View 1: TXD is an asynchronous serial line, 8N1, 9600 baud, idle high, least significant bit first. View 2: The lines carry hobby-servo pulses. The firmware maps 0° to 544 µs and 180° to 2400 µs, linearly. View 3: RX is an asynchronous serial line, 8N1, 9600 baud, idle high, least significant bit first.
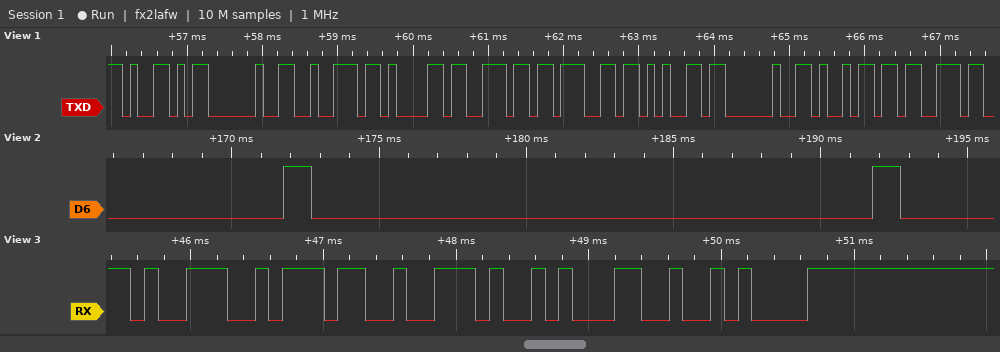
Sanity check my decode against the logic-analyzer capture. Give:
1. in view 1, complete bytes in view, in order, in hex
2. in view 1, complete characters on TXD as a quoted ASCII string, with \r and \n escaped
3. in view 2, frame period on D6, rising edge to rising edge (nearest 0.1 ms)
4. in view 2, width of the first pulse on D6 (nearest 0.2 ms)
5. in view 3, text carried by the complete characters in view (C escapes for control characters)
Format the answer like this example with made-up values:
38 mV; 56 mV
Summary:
59 20 72 61 6E 67 65 20 69 73; "Y range is"; 20.0 ms; 1.0 ms; "97.1\n"
